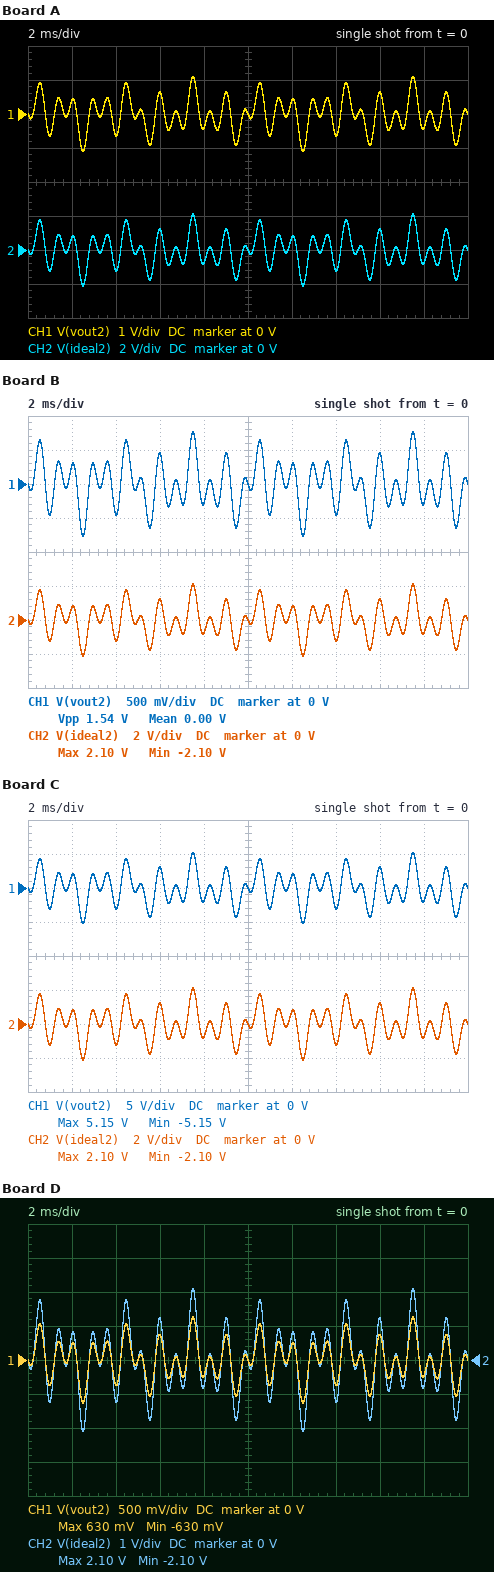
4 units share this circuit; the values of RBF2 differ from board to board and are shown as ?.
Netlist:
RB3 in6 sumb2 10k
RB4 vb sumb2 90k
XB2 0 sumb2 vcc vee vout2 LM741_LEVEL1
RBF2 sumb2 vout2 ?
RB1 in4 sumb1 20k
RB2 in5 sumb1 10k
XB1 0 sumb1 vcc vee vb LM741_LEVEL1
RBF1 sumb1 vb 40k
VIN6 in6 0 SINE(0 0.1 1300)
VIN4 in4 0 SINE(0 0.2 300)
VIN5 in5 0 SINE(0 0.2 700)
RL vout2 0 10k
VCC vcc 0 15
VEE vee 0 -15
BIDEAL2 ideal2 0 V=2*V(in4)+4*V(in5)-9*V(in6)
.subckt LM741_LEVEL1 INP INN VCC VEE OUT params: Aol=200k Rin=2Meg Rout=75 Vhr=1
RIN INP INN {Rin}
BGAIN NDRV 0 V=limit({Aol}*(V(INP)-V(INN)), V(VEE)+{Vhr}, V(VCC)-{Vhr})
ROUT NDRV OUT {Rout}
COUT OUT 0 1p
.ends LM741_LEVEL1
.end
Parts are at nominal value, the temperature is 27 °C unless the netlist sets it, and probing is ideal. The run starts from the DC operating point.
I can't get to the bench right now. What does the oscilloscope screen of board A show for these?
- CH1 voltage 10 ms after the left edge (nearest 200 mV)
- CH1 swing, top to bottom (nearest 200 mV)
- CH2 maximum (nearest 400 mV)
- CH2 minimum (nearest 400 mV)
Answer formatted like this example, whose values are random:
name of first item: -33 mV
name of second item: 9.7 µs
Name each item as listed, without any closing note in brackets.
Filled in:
CH1 voltage 10 ms after the left edge: 0 V
CH1 swing, top to bottom: 2.2 V
CH2 maximum: 2.0 V
CH2 minimum: -2.0 V
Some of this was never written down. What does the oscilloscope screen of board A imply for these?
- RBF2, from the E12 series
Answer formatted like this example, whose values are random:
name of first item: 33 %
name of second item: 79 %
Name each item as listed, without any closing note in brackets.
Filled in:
RBF2, from the E12 series: 47 kΩ
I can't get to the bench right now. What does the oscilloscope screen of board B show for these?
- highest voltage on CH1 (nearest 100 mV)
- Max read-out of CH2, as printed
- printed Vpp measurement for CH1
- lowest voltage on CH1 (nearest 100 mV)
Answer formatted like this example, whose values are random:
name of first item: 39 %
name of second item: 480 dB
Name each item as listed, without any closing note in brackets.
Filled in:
highest voltage on CH1: 800 mV
Max read-out of CH2, as printed: 2.10 V
printed Vpp measurement for CH1: 1.54 V
lowest voltage on CH1: -800 mV
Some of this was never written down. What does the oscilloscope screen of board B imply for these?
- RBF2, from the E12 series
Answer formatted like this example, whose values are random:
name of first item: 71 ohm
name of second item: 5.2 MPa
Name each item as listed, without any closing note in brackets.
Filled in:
RBF2, from the E12 series: 33 kΩ
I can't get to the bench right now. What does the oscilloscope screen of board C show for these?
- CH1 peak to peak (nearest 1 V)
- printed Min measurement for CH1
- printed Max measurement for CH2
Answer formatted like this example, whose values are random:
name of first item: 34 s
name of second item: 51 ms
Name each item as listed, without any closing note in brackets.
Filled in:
CH1 peak to peak: 10 V
printed Min measurement for CH1: -5.15 V
printed Max measurement for CH2: 2.10 V
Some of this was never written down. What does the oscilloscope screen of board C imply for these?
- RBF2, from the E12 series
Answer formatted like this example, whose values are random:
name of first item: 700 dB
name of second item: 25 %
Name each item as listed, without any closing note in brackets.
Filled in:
RBF2, from the E12 series: 220 kΩ
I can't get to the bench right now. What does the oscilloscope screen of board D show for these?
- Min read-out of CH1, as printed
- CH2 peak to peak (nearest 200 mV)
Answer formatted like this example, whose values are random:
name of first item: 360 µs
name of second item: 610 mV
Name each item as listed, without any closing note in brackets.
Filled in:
Min read-out of CH1, as printed: -630 mV
CH2 peak to peak: 4.2 V
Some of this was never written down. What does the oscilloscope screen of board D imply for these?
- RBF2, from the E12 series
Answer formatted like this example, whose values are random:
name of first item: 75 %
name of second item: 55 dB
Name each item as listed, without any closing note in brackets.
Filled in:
RBF2, from the E12 series: 27 kΩ
